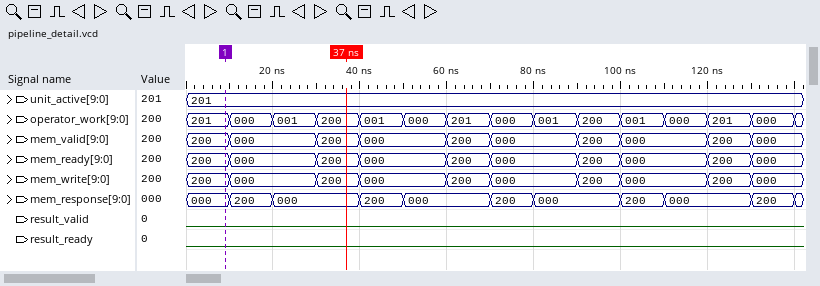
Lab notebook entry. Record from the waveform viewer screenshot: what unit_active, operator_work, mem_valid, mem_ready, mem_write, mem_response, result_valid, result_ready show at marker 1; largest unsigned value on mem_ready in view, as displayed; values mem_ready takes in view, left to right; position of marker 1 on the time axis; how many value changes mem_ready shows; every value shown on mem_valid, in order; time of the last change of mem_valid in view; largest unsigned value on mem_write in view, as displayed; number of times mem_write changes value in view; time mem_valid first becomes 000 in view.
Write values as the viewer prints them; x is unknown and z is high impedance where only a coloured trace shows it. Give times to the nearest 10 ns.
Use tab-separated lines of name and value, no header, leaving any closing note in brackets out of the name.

what unit_active, operator_work, mem_valid, mem_ready, mem_write, mem_response, result_valid, result_ready show at marker 1	unit_active=201, operator_work=201, mem_valid=200, mem_ready=200, mem_write=200, mem_response=000, result_valid=0, result_ready=0
largest unsigned value on mem_ready in view, as displayed	200
values mem_ready takes in view, left to right	200, 000, 200, 000, 200, 000, 200, 000, 200, 000
position of marker 1 on the time axis	10 ns
how many value changes mem_ready shows	9
every value shown on mem_valid, in order	200, 000, 200, 000, 200, 000, 200, 000, 200, 000
time of the last change of mem_valid in view	130 ns
largest unsigned value on mem_write in view, as displayed	200
number of times mem_write changes value in view	9
time mem_valid first becomes 000 in view	10 ns
